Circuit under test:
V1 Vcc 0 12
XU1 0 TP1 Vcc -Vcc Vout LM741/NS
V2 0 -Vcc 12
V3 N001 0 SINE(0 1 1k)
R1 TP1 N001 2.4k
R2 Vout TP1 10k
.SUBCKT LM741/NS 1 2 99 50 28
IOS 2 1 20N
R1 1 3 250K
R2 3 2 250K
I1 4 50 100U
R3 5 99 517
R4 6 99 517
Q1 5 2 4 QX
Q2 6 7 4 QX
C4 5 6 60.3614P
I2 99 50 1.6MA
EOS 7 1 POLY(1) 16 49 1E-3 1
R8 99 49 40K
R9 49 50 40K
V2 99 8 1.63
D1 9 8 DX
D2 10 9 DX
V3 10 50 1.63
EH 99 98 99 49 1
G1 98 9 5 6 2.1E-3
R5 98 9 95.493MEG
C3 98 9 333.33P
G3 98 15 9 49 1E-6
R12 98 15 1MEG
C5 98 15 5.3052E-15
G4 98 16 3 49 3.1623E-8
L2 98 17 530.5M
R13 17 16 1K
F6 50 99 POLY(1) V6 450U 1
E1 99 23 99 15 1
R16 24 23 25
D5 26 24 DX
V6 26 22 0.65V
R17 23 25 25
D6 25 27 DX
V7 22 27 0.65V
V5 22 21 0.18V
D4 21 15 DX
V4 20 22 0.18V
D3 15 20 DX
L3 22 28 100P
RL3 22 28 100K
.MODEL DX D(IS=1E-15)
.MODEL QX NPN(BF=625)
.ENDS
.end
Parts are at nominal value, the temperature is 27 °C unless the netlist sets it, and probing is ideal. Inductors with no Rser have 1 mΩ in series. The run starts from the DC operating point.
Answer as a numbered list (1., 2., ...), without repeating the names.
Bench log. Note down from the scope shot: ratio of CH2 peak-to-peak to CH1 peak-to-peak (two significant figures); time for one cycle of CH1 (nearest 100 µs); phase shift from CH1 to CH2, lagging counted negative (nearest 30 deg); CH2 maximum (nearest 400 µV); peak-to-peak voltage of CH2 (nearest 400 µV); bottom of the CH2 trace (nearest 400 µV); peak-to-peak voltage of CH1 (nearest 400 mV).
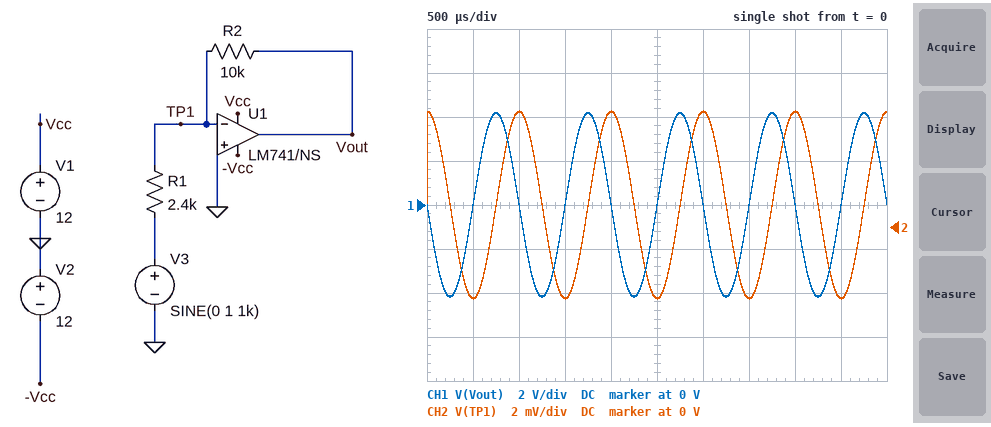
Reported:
1. 0.0010
2. 1.0 ms
3. -90 deg
4. 5.2 mV
5. 8.4 mV
6. -3.2 mV
7. 8.4 V
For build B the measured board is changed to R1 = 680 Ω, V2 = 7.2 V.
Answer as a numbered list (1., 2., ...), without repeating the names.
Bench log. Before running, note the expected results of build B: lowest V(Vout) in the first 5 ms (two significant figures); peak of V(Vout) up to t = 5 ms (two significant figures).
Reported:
1. -6.2 V
2. 11 V
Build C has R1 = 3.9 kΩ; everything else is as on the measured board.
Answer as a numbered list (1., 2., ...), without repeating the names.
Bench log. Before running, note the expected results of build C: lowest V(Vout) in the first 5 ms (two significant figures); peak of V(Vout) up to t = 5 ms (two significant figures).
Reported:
1. -2.6 V
2. 2.6 V
